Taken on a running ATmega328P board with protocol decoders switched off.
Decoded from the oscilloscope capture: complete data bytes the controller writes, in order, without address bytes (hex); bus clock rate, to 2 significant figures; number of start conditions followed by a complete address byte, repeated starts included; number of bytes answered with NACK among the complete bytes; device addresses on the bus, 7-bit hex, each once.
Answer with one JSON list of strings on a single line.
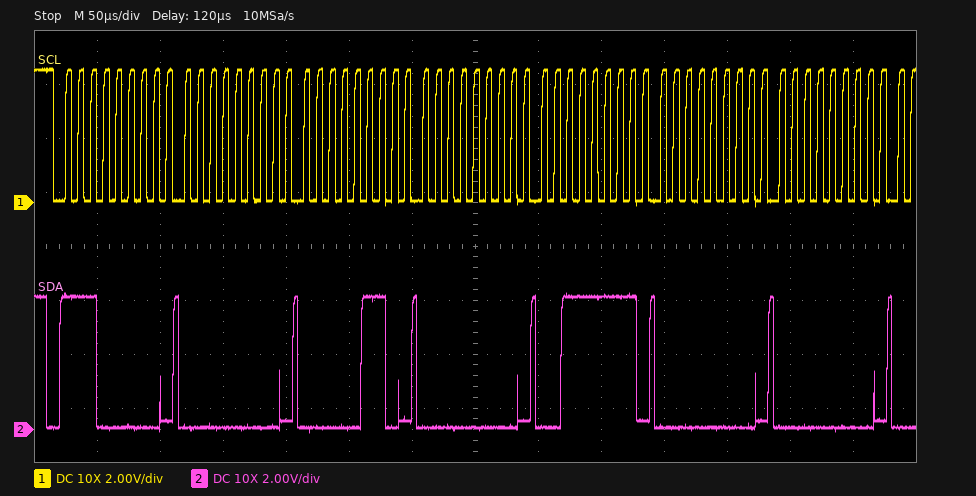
["00 06 00 3F 00 00", "100 kHz", "1", "0", "0x70"]
